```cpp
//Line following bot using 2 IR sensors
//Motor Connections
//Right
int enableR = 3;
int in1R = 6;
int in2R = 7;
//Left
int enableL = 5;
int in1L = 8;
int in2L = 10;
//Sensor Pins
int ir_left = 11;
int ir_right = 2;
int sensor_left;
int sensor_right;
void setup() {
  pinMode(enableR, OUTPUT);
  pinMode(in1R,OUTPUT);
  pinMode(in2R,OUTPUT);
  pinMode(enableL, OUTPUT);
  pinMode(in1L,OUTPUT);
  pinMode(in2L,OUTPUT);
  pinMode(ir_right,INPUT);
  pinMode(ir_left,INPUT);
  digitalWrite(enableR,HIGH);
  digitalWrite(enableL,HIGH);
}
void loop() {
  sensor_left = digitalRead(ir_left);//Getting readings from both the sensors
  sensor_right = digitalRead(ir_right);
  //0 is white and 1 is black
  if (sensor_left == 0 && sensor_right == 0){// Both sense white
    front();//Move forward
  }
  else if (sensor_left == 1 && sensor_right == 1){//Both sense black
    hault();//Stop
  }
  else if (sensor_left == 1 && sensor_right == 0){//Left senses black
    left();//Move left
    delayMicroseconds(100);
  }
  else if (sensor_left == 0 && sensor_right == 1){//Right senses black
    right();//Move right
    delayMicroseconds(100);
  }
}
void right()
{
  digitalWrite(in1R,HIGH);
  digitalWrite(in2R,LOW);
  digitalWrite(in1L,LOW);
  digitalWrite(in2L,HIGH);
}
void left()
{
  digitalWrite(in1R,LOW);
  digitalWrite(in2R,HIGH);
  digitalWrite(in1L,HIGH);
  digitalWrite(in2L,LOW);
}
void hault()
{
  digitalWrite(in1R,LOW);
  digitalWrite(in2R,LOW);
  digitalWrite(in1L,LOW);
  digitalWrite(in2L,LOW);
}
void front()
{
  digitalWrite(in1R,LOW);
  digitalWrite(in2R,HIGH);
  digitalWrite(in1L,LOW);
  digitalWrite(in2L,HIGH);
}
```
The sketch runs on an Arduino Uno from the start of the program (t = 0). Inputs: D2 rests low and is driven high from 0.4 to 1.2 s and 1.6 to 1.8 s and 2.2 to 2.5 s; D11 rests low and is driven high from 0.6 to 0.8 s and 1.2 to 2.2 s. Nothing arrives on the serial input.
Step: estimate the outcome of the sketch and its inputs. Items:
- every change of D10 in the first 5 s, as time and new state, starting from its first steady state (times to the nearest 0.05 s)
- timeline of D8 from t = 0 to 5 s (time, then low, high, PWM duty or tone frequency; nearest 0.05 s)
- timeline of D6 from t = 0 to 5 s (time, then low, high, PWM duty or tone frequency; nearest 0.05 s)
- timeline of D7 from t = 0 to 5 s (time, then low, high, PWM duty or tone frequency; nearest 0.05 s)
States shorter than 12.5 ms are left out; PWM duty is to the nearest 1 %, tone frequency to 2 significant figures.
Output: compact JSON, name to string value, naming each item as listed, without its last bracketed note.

{"every change of D10 in the first 5 s, as time and new state, starting from its first steady state": "0 s high; 0.6 s low; 0.8 s high; 1.2 s low; 2.2 s high", "timeline of D8 from t = 0 to 5 s": "0 s low; 1.2 s high; 1.6 s low; 1.8 s high; 2.2 s low", "timeline of D6 from t = 0 to 5 s": "0 s low; 0.4 s high; 0.6 s low; 0.8 s high; 1.2 s low; 2.2 s high; 2.5 s low", "timeline of D7 from t = 0 to 5 s": "0 s high; 0.4 s low; 1.2 s high; 1.6 s low; 1.8 s high; 2.2 s low; 2.5 s high"}
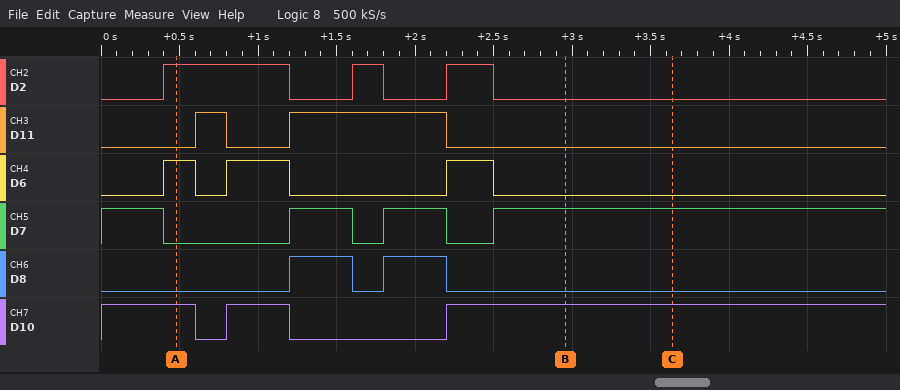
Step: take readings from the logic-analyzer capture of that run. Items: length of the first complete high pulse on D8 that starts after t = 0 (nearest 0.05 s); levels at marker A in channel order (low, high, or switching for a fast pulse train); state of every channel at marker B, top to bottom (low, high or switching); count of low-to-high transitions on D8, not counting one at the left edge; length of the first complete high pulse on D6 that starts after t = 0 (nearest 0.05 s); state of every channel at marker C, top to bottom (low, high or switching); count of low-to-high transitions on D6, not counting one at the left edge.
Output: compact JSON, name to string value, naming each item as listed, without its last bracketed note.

{"length of the first complete high pulse on D8 that starts after t = 0": "0.40 s", "levels at marker A in channel order": "D2 high, D11 low, D6 high, D7 low, D8 low, D10 high", "state of every channel at marker B, top to bottom": "D2 low, D11 low, D6 low, D7 high, D8 low, D10 high", "count of low-to-high transitions on D8, not counting one at the left edge": "2", "length of the first complete high pulse on D6 that starts after t = 0": "0.20 s", "state of every channel at marker C, top to bottom": "D2 low, D11 low, D6 low, D7 high, D8 low, D10 high", "count of low-to-high transitions on D6, not counting one at the left edge": "3"}
